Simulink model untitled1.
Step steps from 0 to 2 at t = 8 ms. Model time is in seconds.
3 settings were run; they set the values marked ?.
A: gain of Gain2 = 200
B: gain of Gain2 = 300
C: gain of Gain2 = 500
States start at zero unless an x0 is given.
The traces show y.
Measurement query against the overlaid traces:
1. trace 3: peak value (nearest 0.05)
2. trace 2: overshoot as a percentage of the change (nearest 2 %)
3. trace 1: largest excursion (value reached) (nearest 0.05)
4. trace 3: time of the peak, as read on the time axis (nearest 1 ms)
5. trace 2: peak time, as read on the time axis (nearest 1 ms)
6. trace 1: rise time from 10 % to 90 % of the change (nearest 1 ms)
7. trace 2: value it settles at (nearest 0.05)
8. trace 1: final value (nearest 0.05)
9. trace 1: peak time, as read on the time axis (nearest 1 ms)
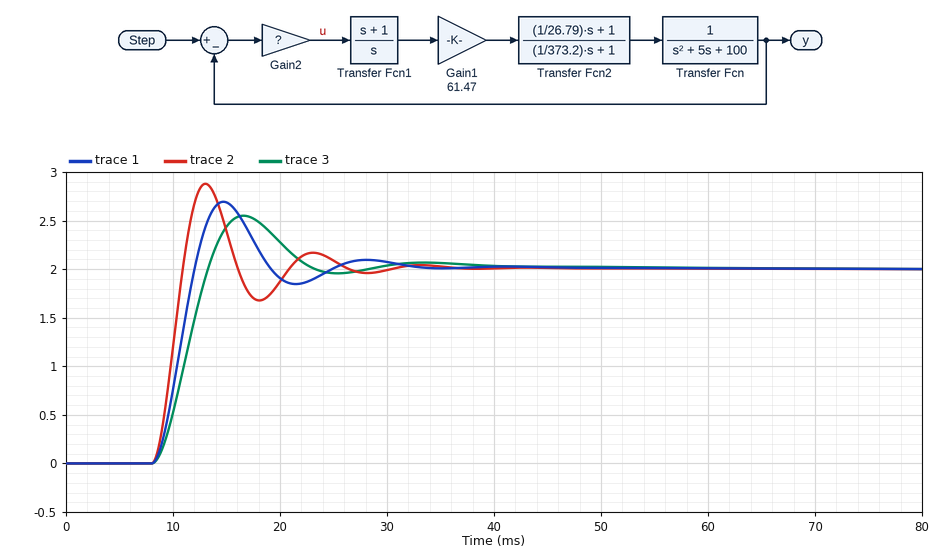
2.55
44 %
2.70
17 ms
13 ms
3 ms
2.00
2.00
15 ms
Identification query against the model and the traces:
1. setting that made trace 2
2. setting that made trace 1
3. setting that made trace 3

C
B
A
